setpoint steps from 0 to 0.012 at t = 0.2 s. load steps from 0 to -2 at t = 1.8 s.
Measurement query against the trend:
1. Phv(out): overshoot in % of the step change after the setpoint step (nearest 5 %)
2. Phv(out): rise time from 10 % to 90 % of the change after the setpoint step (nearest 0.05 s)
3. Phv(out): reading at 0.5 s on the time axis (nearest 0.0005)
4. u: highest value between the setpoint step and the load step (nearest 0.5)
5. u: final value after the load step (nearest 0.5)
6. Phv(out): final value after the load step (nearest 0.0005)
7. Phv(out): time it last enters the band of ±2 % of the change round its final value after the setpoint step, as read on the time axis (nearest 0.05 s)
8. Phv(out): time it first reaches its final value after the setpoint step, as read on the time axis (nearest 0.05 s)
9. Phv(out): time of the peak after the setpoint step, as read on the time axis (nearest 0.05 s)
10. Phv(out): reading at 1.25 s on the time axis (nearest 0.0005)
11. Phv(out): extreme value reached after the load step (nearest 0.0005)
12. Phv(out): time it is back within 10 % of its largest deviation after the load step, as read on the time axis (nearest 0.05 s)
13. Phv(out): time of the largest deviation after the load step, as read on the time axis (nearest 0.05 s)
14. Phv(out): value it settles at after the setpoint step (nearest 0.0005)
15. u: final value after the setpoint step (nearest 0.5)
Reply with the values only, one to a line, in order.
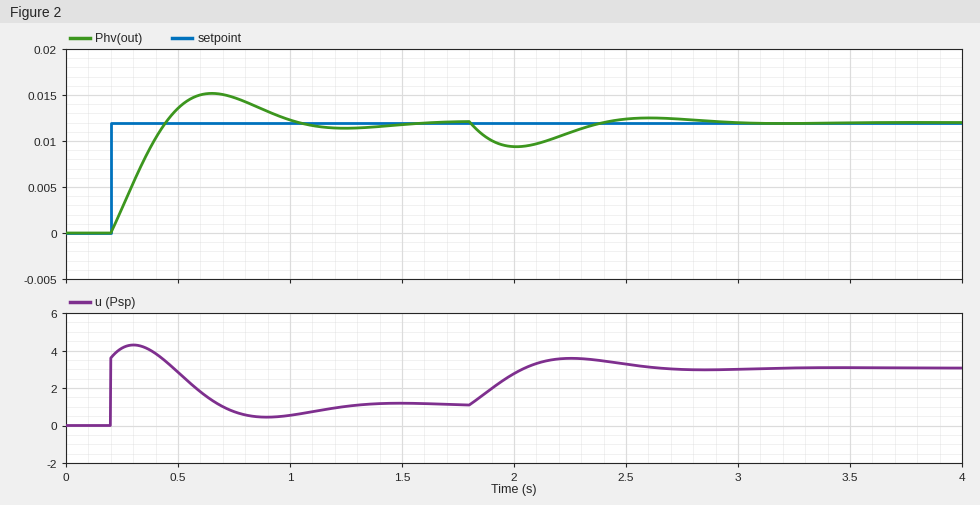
25 %
0.20 s
0.0135
4.5
3.0
0.0120
1.50 s
0.45 s
0.65 s
0.0115
0.0095
2.80 s
2.00 s
0.0120
1.0
